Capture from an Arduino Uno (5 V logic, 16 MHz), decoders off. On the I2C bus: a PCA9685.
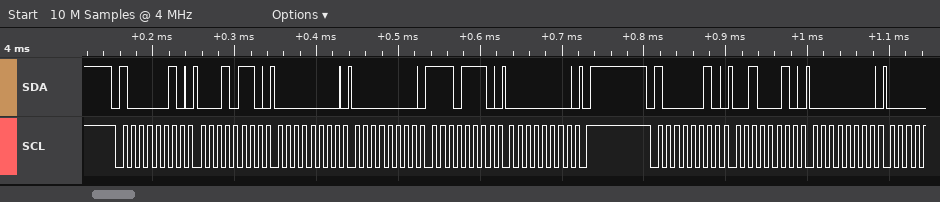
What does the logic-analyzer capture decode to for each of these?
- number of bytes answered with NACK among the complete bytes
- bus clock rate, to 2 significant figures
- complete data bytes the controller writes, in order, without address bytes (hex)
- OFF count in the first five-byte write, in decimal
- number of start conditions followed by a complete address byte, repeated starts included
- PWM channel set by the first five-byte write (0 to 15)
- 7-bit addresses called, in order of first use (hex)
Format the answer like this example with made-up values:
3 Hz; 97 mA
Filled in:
0; 100 kHz; 16 00 00 EE 00 22 00; 238; 2; 4; 0x41
